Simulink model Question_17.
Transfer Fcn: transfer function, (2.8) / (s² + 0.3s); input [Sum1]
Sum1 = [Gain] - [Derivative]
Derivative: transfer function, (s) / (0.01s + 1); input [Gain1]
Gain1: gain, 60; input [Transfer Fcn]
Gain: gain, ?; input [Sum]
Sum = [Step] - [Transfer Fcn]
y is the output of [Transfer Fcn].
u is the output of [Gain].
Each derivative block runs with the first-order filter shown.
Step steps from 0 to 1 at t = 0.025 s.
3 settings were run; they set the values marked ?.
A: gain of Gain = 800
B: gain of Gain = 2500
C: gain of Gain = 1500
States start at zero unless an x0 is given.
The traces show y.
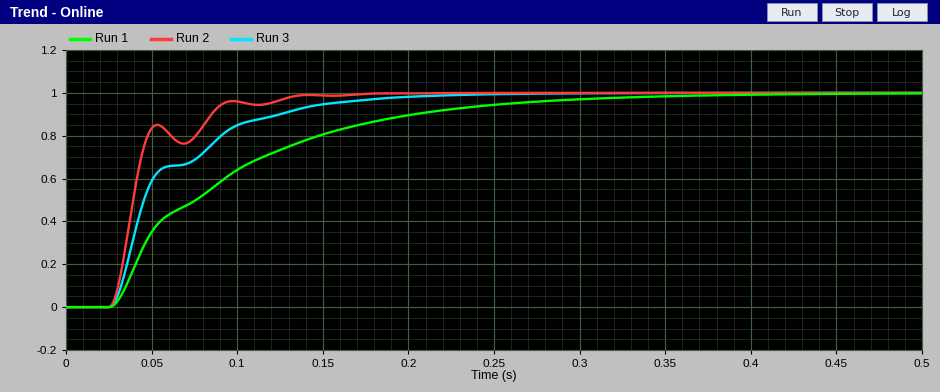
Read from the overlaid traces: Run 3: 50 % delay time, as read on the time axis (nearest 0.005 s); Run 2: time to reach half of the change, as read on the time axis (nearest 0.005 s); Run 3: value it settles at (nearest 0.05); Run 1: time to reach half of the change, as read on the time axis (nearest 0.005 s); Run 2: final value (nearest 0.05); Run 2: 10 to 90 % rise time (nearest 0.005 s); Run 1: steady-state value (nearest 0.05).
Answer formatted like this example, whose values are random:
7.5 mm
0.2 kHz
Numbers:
0.045 s
0.040 s
1.00
0.075 s
1.00
0.055 s
1.00
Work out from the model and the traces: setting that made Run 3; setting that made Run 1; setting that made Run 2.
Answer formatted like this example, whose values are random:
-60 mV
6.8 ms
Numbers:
C
A
B
